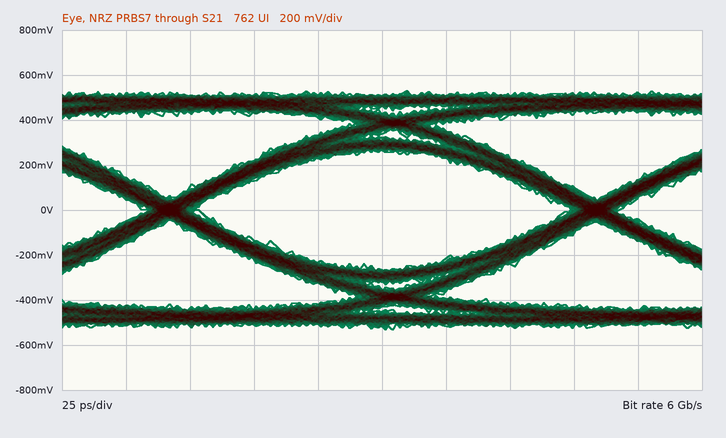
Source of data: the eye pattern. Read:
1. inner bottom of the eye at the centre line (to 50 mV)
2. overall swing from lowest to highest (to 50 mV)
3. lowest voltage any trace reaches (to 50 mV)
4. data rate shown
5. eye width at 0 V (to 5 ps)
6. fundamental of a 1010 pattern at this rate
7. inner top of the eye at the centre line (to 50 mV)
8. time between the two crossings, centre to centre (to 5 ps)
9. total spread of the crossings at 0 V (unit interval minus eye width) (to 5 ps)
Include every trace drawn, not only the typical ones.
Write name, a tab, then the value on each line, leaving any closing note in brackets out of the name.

inner bottom of the eye at the centre line	-250 mV
overall swing from lowest to highest	1.05 V
lowest voltage any trace reaches	-550 mV
data rate shown	6 Gb/s
eye width at 0 V	145 ps
fundamental of a 1010 pattern at this rate	3 GHz
inner top of the eye at the centre line	250 mV
time between the two crossings, centre to centre	165 ps
total spread of the crossings at 0 V (unit interval minus eye width)	20 ps
